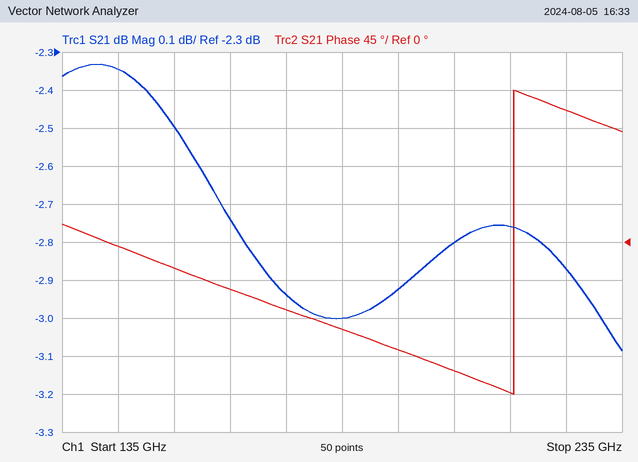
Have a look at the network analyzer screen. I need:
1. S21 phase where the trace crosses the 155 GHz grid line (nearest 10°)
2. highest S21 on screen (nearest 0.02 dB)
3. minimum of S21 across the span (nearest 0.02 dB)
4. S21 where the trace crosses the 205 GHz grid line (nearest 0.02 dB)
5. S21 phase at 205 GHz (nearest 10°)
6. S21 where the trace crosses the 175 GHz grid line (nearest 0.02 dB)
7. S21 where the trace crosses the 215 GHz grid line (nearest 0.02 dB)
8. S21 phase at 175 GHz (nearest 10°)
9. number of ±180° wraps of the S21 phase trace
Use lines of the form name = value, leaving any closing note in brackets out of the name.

S21 phase where the trace crosses the 155 GHz grid line = -30°
highest S21 on screen = -2.34 dB
minimum of S21 across the span = -3.08 dB
S21 where the trace crosses the 205 GHz grid line = -2.80 dB
S21 phase at 205 GHz = -150°
S21 where the trace crosses the 175 GHz grid line = -2.94 dB
S21 where the trace crosses the 215 GHz grid line = -2.76 dB
S21 phase at 175 GHz = -80°
number of ±180° wraps of the S21 phase trace = 1
